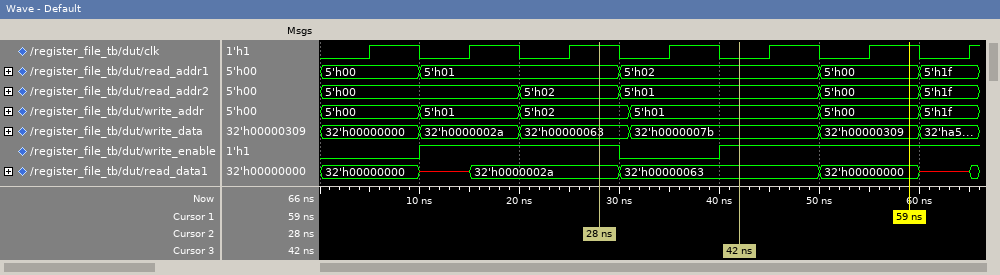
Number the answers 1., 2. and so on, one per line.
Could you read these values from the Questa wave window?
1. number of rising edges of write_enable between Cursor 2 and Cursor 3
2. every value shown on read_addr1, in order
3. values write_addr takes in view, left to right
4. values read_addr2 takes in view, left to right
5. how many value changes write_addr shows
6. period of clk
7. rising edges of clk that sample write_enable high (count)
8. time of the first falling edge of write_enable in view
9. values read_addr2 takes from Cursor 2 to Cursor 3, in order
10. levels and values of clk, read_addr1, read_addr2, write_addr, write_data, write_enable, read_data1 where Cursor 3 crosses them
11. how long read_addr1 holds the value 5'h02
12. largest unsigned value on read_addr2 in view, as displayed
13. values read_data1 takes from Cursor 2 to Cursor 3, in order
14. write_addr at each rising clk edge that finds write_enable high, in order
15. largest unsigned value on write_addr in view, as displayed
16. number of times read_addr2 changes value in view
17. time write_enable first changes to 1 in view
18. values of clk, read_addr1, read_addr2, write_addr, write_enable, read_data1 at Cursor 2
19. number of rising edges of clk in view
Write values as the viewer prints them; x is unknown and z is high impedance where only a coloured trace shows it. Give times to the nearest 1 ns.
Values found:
1. 1
2. 5'h00, 5'h01, 5'h02, 5'h00, 5'h1f
3. 5'h00, 5'h01, 5'h02, 5'h01, 5'h00, 5'h1f
4. 5'h00, 5'h02, 5'h01, 5'h00, 5'h1f
5. 5
6. 10 ns
7. 5
8. 30 ns
9. 5'h02, 5'h01
10. clk=0, read_addr1=5'h02, read_addr2=5'h01, write_addr=5'h01, write_data=32'h0000007b, write_enable=1, read_data1=32'h00000063
11. 20 ns
12. 5'h1f
13. 32'h0000002a, 32'h00000063
14. 5'h01, 5'h02, 5'h01, 5'h00, 5'h1f
15. 5'h1f
16. 4
17. 10 ns
18. clk=1, read_addr1=5'h01, read_addr2=5'h02, write_addr=5'h02, write_enable=1, read_data1=32'h0000002a
19. 7
